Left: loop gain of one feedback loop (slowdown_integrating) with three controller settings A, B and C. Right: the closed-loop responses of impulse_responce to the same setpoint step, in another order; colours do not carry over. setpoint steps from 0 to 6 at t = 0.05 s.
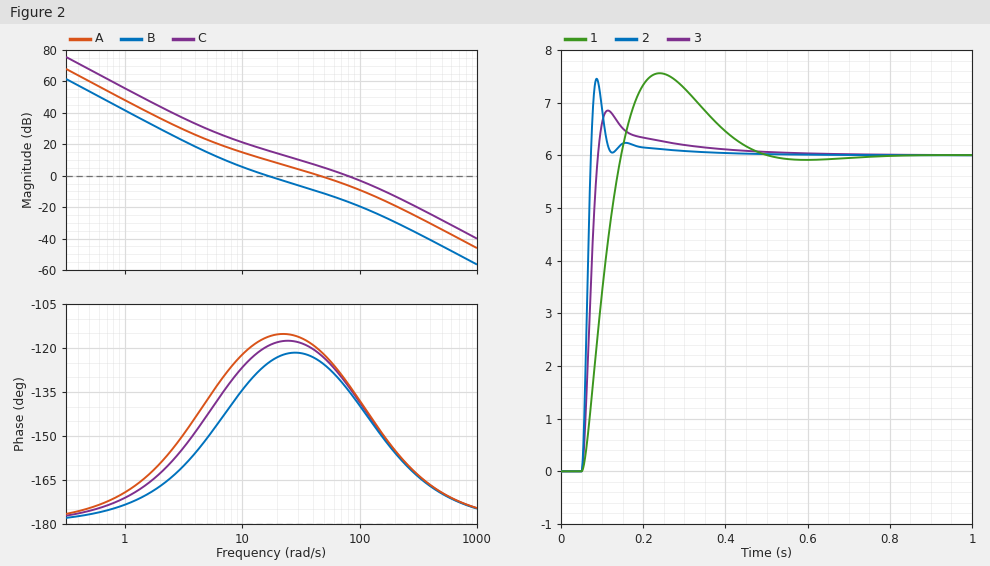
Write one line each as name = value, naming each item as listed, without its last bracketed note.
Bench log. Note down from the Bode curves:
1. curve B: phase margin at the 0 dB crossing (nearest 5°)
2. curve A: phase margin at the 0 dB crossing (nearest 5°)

curve B: phase margin at the 0 dB crossing = 55°
curve A: phase margin at the 0 dB crossing = 60°
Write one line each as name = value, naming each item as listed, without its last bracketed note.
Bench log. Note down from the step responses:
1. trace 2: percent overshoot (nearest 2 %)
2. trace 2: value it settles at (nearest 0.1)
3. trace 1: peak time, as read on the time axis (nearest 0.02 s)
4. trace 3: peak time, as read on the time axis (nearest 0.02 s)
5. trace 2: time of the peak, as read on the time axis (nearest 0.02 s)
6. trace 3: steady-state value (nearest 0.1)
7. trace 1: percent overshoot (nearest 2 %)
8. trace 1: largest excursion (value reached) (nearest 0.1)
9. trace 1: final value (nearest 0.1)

trace 2: percent overshoot = 24 %
trace 2: value it settles at = 6.0
trace 1: peak time, as read on the time axis = 0.24 s
trace 3: peak time, as read on the time axis = 0.12 s
trace 2: time of the peak, as read on the time axis = 0.08 s
trace 3: steady-state value = 6.0
trace 1: percent overshoot = 26 %
trace 1: largest excursion (value reached) = 7.6
trace 1: final value = 6.0
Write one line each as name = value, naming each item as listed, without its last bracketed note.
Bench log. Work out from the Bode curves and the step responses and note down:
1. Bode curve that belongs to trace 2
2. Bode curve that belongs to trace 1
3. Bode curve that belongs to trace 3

Bode curve that belongs to trace 2 = C
Bode curve that belongs to trace 1 = B
Bode curve that belongs to trace 3 = A
